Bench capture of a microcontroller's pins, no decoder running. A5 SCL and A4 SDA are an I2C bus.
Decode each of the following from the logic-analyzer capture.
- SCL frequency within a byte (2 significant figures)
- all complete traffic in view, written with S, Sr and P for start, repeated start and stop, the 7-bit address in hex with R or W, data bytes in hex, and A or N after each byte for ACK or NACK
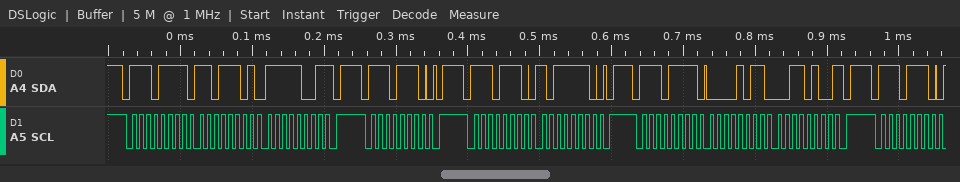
100 kHz
S 77R A DD A F9 N P S 77W A P S 77W A BE A P S 77R A 0B A 34 N P S 77W A
